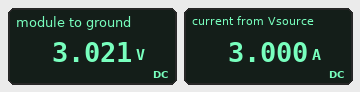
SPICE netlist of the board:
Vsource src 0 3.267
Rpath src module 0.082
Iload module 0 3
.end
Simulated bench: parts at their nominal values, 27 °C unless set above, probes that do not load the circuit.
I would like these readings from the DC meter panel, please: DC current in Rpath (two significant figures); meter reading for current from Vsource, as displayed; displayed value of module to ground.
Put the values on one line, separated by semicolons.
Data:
3.0 A; 3.000 A; 3.021 V
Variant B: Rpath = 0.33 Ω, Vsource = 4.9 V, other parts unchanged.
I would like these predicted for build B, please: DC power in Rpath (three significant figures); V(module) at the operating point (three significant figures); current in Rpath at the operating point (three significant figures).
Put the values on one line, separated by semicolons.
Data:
2.97 W; 3.91 V; 3.00 A
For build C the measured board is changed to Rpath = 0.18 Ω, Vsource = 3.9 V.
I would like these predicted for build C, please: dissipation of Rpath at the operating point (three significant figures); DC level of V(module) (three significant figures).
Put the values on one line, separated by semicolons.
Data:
1.62 W; 3.36 V
